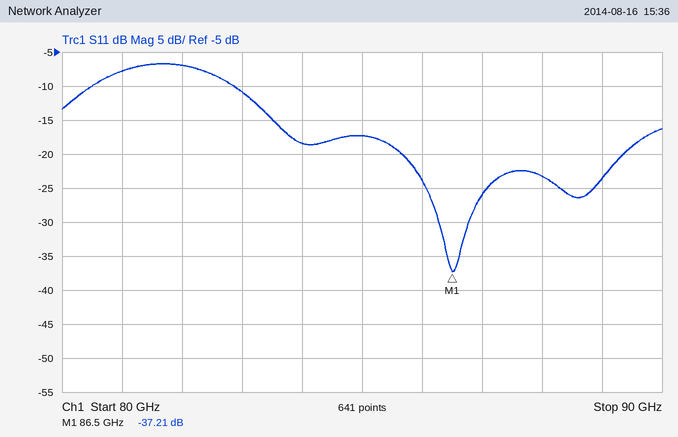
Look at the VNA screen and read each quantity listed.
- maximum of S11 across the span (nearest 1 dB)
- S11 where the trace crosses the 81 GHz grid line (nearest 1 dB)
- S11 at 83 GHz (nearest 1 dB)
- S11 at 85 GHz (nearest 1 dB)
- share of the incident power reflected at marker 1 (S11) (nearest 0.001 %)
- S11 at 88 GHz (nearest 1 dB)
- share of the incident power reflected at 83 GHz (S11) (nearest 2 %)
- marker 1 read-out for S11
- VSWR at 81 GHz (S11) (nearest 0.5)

-7 dB
-8 dB
-11 dB
-17 dB
0.019 %
-23 dB
8 %
-37.21 dB
2.5
